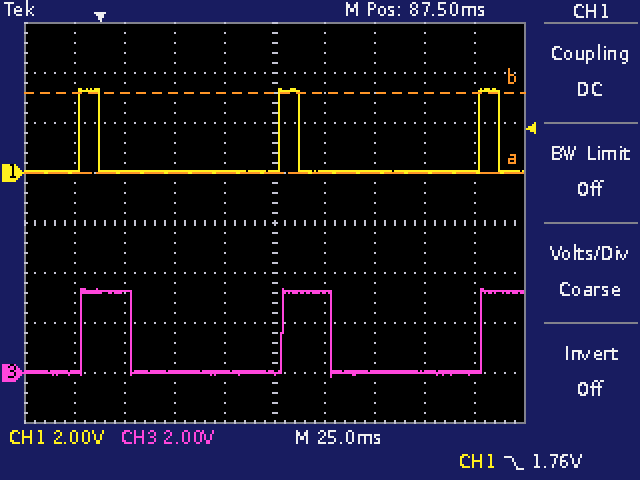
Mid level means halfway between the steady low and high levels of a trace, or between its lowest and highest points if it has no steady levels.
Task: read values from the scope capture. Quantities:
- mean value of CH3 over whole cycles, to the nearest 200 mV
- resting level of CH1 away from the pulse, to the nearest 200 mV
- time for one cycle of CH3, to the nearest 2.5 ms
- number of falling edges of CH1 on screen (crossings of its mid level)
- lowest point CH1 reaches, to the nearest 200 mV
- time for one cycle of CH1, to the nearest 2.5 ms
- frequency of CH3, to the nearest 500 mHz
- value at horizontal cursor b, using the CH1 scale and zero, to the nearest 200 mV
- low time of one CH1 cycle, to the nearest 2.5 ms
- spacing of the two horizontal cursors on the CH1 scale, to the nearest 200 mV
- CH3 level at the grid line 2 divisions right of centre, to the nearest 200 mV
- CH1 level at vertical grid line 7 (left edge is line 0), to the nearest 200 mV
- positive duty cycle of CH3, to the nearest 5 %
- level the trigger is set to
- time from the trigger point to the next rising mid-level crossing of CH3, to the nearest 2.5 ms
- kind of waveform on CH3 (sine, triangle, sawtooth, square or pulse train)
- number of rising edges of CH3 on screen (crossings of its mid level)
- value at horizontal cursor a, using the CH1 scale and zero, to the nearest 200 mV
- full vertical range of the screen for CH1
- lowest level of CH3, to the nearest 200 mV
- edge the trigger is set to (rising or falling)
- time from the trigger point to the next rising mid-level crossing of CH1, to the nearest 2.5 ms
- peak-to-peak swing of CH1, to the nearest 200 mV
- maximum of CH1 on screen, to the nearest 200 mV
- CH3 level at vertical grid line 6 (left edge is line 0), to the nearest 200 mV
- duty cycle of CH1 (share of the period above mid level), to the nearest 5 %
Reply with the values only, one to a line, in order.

800 mV
0.0 V
100.0 ms
3
0.0 V
100.0 ms
10.0 Hz
3.2 V
90.0 ms
3.2 V
0.0 V
0.0 V
25 %
1.76 V
92.5 ms
pulse train
3
0.0 V
16 V
-200 mV
falling
90.0 ms
3.4 V
3.4 V
3.2 V
10 %
